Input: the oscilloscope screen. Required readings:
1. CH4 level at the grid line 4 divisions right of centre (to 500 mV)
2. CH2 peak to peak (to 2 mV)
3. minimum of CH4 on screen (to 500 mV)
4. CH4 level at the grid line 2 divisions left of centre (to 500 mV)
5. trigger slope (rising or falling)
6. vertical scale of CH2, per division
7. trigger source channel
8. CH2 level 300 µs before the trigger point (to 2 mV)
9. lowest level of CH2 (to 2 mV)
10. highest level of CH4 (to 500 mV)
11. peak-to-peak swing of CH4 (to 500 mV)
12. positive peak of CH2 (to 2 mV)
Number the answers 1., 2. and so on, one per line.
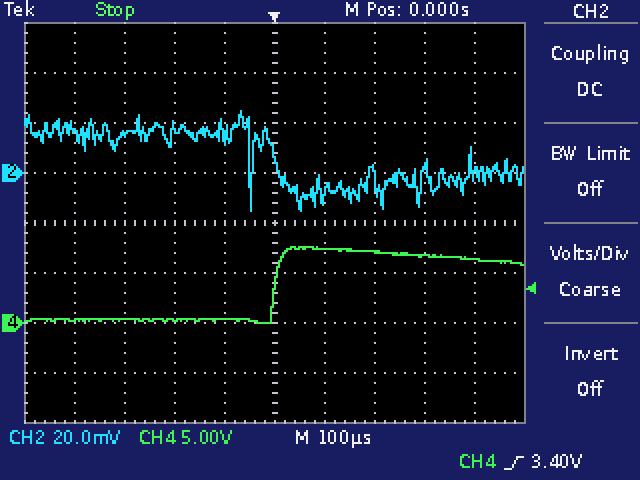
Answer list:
1. 6.5 V
2. 40 mV
3. 0.0 V
4. 500 mV
5. rising
6. 20 mV
7. CH4
8. 16 mV
9. -16 mV
10. 7.5 V
11. 7.5 V
12. 24 mV
